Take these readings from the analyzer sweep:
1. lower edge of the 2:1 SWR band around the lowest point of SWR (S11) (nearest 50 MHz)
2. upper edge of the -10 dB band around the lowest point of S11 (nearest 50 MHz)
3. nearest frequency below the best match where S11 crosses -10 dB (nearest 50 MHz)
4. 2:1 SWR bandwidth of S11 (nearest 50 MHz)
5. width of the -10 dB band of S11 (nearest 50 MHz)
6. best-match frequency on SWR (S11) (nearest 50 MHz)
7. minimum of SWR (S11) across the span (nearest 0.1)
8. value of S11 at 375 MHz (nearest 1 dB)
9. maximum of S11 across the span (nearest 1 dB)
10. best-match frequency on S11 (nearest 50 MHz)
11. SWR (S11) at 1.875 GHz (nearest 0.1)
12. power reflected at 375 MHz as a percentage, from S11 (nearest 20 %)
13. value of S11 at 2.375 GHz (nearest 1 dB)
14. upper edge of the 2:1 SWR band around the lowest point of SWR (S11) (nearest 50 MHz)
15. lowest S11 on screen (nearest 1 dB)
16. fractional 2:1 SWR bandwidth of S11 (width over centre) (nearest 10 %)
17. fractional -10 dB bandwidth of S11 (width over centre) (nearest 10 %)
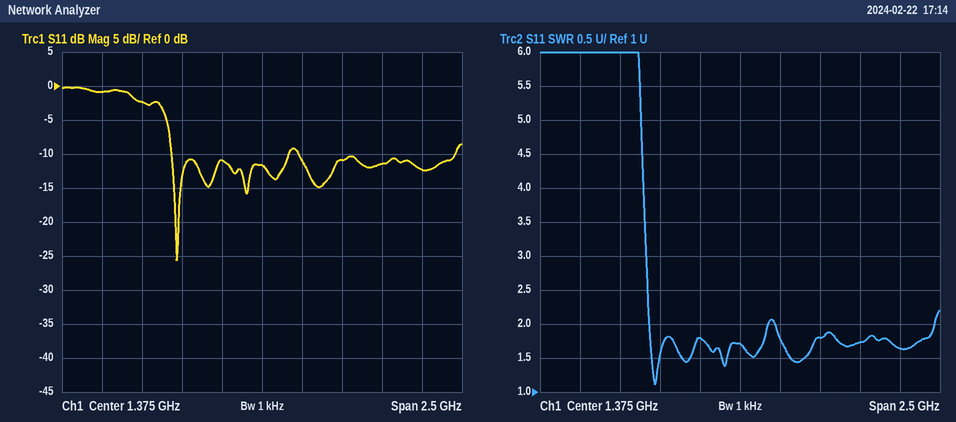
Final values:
800 MHz
1.55 GHz
800 MHz
750 MHz
750 MHz
850 MHz
1.1
-1 dB
0 dB
850 MHz
1.8
80 %
-12 dB
1.55 GHz
-26 dB
60 %
60 %
